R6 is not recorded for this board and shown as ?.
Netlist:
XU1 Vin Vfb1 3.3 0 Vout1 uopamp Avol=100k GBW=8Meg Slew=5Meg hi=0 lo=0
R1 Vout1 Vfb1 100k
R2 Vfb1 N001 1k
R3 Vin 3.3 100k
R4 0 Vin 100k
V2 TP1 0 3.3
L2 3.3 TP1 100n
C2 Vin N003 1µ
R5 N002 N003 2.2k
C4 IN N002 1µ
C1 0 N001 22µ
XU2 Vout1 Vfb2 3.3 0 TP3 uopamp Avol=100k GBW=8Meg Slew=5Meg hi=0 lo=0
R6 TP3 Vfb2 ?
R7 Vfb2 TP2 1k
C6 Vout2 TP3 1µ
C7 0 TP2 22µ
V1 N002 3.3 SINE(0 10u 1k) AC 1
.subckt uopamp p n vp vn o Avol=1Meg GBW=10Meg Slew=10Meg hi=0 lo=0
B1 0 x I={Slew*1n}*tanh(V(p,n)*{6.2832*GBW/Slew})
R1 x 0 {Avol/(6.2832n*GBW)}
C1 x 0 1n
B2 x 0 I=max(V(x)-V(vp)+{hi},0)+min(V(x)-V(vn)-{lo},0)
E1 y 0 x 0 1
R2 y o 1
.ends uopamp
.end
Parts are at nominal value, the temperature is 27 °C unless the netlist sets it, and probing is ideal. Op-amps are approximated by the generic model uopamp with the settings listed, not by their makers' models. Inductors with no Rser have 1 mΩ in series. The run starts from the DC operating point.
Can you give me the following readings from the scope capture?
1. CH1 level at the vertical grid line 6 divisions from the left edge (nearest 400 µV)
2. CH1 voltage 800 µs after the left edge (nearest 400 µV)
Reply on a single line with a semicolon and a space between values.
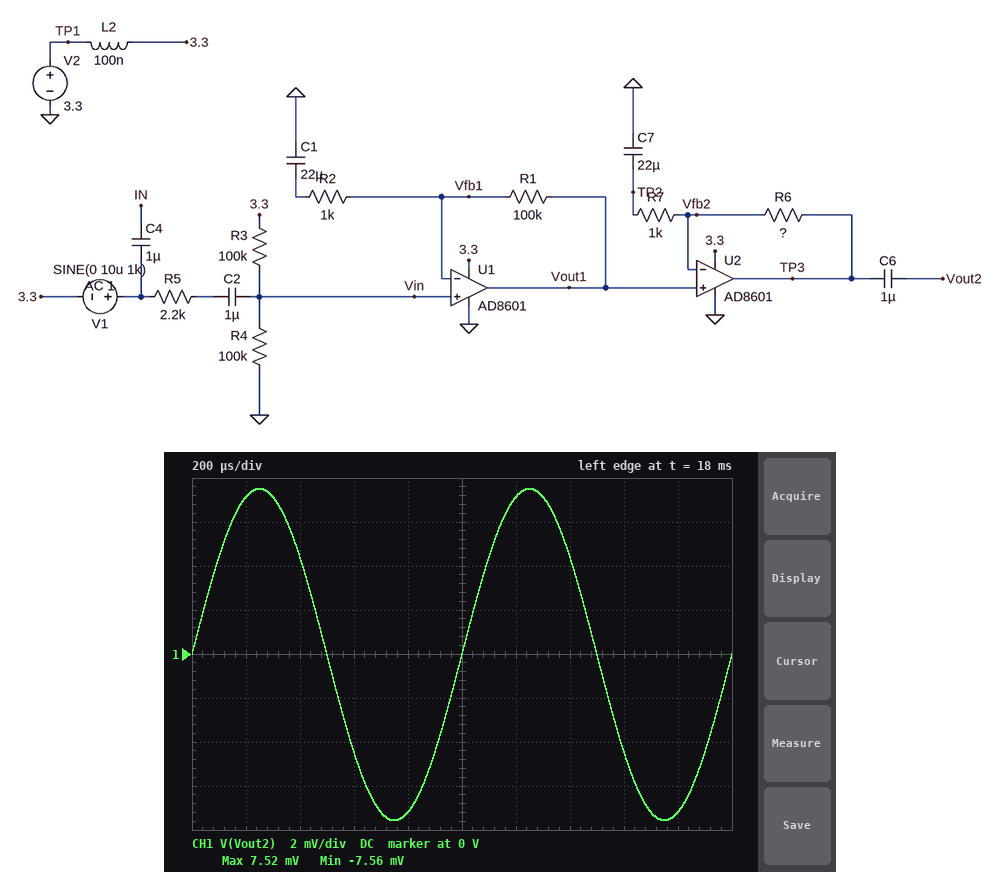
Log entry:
7.2 mV; -7.2 mV
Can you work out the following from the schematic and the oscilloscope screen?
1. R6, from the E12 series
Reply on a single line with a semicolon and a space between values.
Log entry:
6.8 kΩ
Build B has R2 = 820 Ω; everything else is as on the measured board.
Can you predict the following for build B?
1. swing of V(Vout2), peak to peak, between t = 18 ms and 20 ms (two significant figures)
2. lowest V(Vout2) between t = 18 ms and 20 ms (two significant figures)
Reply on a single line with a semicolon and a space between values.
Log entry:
18 mV; -9.2 mV
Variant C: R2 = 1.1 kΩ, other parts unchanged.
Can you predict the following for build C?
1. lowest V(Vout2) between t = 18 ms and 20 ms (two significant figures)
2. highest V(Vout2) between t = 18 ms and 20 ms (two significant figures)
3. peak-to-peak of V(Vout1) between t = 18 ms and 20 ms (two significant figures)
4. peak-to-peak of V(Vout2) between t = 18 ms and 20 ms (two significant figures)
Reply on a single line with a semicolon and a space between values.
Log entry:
-6.9 mV; 6.8 mV; 1.8 mV; 14 mV
